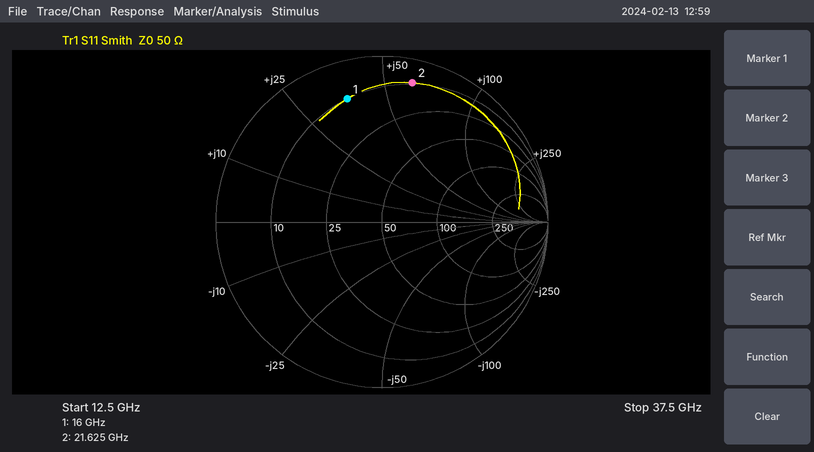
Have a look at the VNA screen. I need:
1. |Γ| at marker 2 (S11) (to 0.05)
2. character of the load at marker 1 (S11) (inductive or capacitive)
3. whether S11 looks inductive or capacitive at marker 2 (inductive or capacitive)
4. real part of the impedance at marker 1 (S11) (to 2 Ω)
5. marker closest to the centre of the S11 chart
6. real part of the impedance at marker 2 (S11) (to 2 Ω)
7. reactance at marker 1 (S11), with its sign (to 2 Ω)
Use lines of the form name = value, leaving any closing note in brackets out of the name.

|Γ| at marker 2 (S11) = 0.85
character of the load at marker 1 (S11) = inductive
whether S11 looks inductive or capacitive at marker 2 = inductive
real part of the impedance at marker 1 (S11) = 10 Ω
marker closest to the centre of the S11 chart = marker 1
real part of the impedance at marker 2 (S11) = 10 Ω
reactance at marker 1 (S11), with its sign = +36 Ω
